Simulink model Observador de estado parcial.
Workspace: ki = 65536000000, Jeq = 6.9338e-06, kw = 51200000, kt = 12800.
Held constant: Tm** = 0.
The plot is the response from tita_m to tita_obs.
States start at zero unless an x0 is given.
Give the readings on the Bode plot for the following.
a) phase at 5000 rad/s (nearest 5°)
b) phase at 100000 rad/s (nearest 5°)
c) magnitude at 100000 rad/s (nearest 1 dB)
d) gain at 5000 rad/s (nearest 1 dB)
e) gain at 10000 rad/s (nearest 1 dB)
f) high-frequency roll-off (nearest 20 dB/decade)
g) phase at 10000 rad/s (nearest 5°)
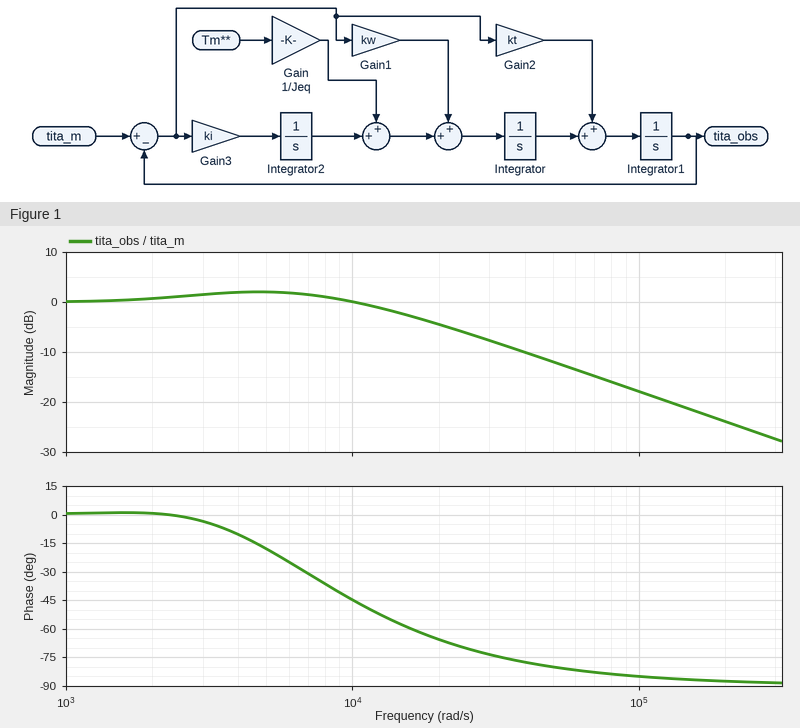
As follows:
-20°
-85°
-18 dB
2 dB
0 dB
-20 dB/decade
-45°
